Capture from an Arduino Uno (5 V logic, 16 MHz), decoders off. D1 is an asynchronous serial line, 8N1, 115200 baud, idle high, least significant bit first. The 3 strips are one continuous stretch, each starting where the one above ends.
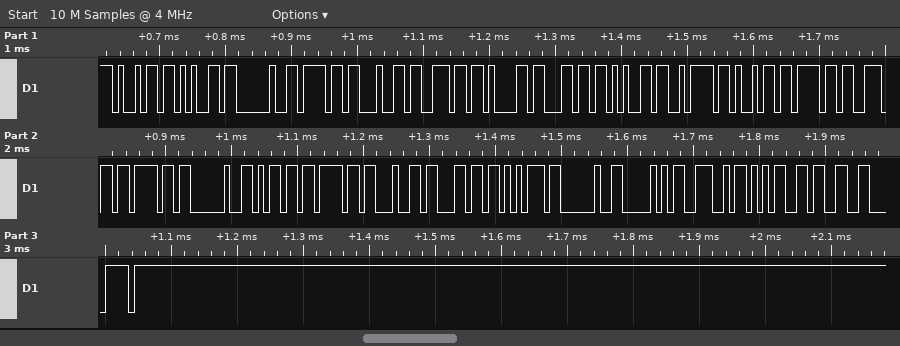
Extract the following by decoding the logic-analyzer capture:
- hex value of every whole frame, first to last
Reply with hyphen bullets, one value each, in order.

- 69 65 20 6F 64 6E 61 6C 65 7A 69 6F 6E 6F 20 6D 6F 64 6C 75 20 50 4E 35 33 78
